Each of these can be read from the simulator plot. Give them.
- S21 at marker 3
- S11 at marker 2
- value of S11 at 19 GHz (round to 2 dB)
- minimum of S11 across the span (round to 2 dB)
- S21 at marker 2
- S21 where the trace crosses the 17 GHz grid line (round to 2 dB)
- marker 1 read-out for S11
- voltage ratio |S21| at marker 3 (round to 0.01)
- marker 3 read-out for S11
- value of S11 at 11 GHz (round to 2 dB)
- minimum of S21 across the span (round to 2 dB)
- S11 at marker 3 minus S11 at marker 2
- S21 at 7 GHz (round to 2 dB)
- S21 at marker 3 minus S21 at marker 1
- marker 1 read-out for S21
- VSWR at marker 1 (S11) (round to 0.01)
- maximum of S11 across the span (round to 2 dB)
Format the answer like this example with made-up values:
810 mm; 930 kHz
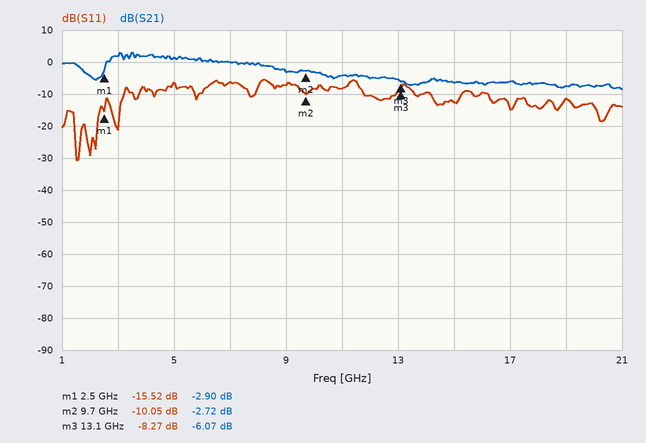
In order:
-6.07 dB; -10.05 dB; -12 dB; -30 dB; -2.72 dB; -6 dB; -15.52 dB; 0.50; -8.27 dB; -8 dB; -8 dB; 1.78 dB; 0 dB; -3.17 dB; -2.90 dB; 1.40; -6 dB
